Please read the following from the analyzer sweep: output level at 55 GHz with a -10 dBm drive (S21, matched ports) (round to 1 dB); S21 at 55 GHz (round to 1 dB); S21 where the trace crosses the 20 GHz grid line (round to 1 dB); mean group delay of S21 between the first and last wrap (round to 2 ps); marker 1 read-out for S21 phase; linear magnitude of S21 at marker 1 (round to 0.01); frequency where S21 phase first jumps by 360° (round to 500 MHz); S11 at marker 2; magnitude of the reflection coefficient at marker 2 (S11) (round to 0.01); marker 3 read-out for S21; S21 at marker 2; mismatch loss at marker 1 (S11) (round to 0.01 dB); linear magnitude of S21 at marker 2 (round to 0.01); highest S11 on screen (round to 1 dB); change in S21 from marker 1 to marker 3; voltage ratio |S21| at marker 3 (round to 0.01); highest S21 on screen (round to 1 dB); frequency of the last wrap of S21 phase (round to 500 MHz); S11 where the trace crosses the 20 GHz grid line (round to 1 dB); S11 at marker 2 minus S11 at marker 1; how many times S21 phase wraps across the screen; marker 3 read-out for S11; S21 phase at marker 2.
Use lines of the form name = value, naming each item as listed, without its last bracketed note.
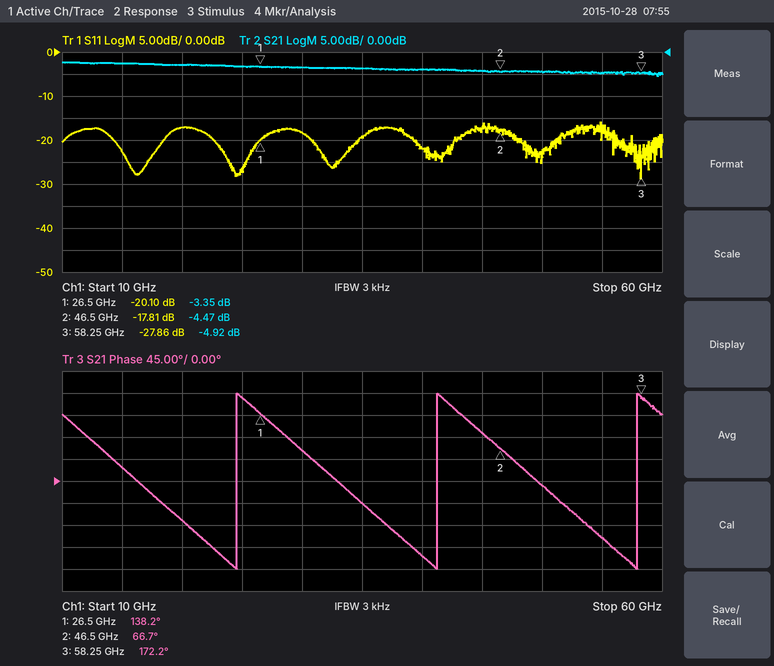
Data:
output level at 55 GHz with a -10 dBm drive (S21, matched ports) = -15 dBm
S21 at 55 GHz = -5 dB
S21 where the trace crosses the 20 GHz grid line = -3 dB
mean group delay of S21 between the first and last wrap = 60 ps
marker 1 read-out for S21 phase = 138.2°
linear magnitude of S21 at marker 1 = 0.68
frequency where S21 phase first jumps by 360° = 24.5 GHz
S11 at marker 2 = -17.81 dB
magnitude of the reflection coefficient at marker 2 (S11) = 0.13
marker 3 read-out for S21 = -4.92 dB
S21 at marker 2 = -4.47 dB
mismatch loss at marker 1 (S11) = 0.04 dB
linear magnitude of S21 at marker 2 = 0.60
highest S11 on screen = -16 dB
change in S21 from marker 1 to marker 3 = -1.57 dB
voltage ratio |S21| at marker 3 = 0.57
highest S21 on screen = -2 dB
frequency of the last wrap of S21 phase = 58.0 GHz
S11 where the trace crosses the 20 GHz grid line = -17 dB
S11 at marker 2 minus S11 at marker 1 = 2.29 dB
how many times S21 phase wraps across the screen = 3
marker 3 read-out for S11 = -27.86 dB
S21 phase at marker 2 = 66.7°
